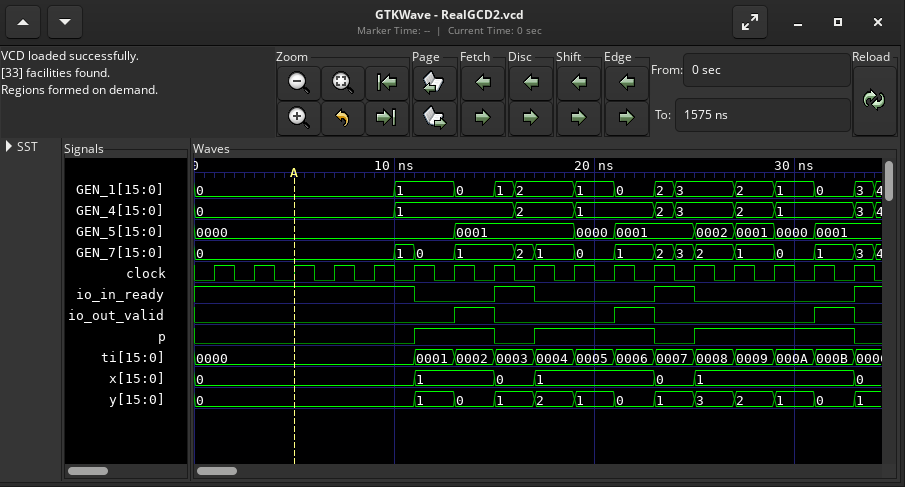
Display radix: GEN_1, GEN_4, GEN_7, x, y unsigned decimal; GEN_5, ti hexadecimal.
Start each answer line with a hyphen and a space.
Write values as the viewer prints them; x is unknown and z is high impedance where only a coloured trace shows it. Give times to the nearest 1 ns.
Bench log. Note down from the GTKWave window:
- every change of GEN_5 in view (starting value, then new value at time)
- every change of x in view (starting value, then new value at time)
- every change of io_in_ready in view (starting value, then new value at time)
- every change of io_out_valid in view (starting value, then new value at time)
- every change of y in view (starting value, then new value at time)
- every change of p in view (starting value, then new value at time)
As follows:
- 0000, 0001 at 13 ns, 0000 at 19 ns, 0001 at 21 ns, 0002 at 25 ns, 0001 at 27 ns, 0000 at 29 ns, 0001 at 31 ns
- 0, 1 at 11 ns, 0 at 15 ns, 1 at 17 ns, 0 at 23 ns, 1 at 25 ns, 0 at 33 ns
- 1, 0 at 11 ns, 1 at 15 ns, 0 at 17 ns, 1 at 23 ns, 0 at 25 ns, 1 at 33 ns
- 0, 1 at 13 ns, 0 at 15 ns, 1 at 21 ns, 0 at 23 ns, 1 at 31 ns, 0 at 33 ns
- 0, 1 at 11 ns, 0 at 13 ns, 1 at 15 ns, 2 at 17 ns, 1 at 19 ns, 0 at 21 ns, 1 at 23 ns, 3 at 25 ns, 2 at 27 ns, 1 at 29 ns, 0 at 31 ns, 1 at 33 ns
- 0, 1 at 11 ns, 0 at 15 ns, 1 at 17 ns, 0 at 23 ns, 1 at 25 ns, 0 at 33 ns
